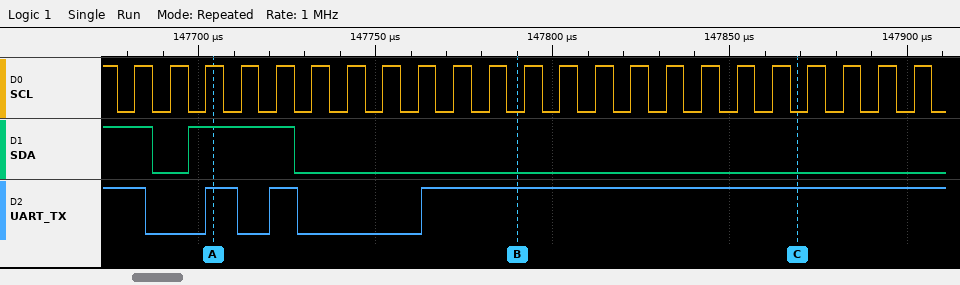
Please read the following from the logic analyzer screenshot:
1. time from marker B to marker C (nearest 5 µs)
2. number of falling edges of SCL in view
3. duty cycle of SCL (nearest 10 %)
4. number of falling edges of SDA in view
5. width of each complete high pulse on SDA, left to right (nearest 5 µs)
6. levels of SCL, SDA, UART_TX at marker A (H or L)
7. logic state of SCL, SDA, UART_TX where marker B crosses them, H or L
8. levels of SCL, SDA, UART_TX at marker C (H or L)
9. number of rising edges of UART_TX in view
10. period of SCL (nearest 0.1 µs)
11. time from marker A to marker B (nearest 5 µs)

80 µs
24
50 %
2
30 µs
SCL=H, SDA=H, UART_TX=H
SCL=L, SDA=L, UART_TX=H
SCL=L, SDA=L, UART_TX=H
3
10 µs
85 µs
